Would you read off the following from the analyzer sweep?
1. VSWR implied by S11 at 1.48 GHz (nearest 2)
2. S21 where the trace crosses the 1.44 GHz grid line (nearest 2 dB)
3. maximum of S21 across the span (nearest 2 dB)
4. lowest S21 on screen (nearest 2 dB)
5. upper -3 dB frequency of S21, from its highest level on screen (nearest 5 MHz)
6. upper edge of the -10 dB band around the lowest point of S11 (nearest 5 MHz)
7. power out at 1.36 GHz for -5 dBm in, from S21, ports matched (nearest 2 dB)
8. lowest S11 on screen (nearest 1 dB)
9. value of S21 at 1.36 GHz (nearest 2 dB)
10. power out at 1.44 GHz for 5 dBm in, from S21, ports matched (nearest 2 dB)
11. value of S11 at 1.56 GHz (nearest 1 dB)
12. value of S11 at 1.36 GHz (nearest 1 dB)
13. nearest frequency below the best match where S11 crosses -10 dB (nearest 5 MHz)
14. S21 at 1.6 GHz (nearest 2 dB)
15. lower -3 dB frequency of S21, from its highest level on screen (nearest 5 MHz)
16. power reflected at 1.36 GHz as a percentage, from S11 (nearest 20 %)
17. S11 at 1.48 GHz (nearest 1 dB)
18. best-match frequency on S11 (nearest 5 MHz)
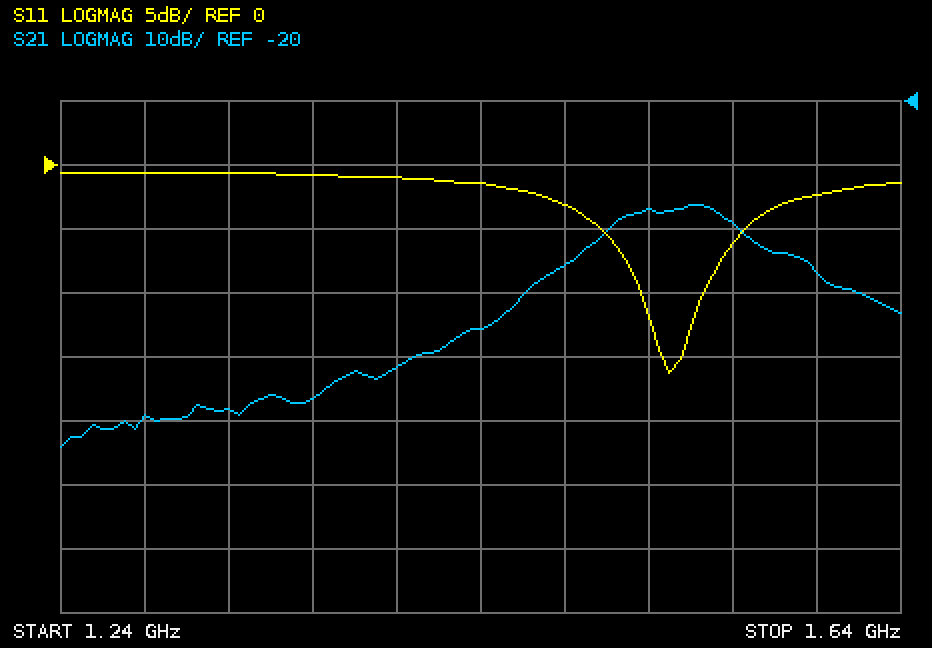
6
-56 dB
-36 dB
-74 dB
1.560 GHz
1.545 GHz
-72 dBm
-16 dB
-66 dB
-50 dBm
-6 dB
-1 dB
1.515 GHz
-46 dB
1.505 GHz
80 %
-3 dB
1.530 GHz
